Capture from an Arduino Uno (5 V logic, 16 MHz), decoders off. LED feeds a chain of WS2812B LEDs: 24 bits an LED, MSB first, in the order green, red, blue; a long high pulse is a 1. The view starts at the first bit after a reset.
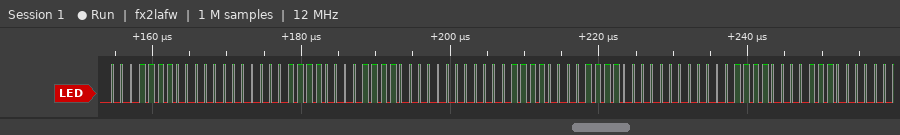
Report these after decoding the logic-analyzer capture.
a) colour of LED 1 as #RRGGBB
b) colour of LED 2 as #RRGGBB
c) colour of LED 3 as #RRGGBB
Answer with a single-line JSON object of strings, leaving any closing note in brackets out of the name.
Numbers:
{"colour of LED 1 as #RRGGBB": "#001E1E", "colour of LED 2 as #RRGGBB": "#001E1E", "colour of LED 3 as #RRGGBB": "#001E1E"}
